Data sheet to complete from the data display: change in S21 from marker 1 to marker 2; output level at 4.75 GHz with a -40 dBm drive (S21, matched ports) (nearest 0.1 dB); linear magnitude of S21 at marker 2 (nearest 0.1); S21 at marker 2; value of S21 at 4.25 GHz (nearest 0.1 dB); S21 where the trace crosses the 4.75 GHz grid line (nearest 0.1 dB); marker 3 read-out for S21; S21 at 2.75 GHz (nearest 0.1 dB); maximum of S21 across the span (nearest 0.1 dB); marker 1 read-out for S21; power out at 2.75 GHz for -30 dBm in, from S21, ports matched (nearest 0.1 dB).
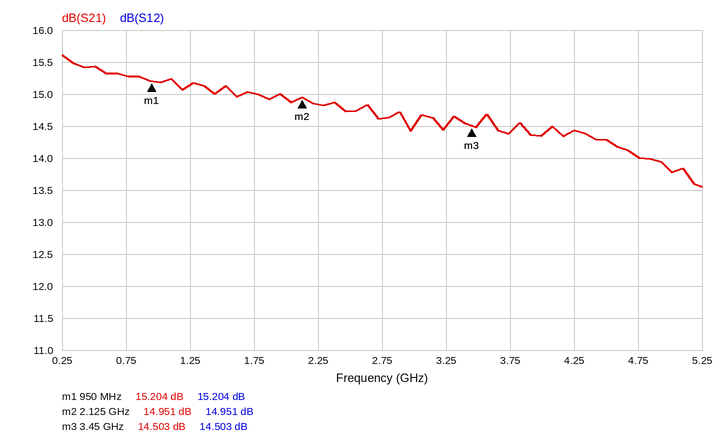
-0.253 dB
-26.0 dBm
5.6
14.951 dB
14.4 dB
14.0 dB
14.503 dB
14.6 dB
15.6 dB
15.204 dB
-15.4 dBm
